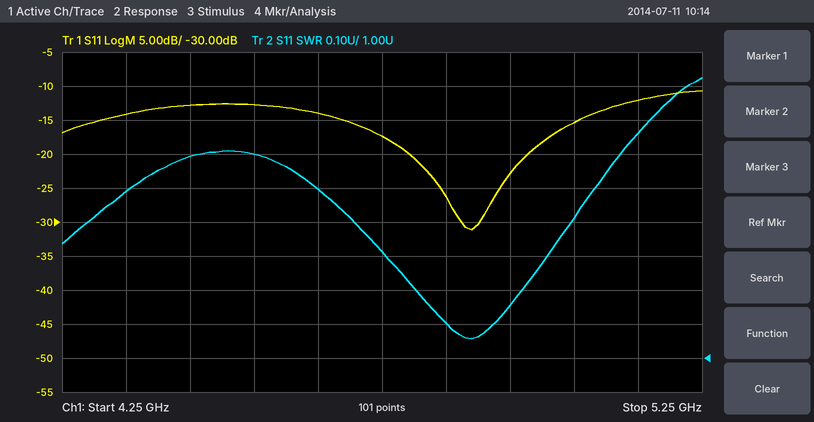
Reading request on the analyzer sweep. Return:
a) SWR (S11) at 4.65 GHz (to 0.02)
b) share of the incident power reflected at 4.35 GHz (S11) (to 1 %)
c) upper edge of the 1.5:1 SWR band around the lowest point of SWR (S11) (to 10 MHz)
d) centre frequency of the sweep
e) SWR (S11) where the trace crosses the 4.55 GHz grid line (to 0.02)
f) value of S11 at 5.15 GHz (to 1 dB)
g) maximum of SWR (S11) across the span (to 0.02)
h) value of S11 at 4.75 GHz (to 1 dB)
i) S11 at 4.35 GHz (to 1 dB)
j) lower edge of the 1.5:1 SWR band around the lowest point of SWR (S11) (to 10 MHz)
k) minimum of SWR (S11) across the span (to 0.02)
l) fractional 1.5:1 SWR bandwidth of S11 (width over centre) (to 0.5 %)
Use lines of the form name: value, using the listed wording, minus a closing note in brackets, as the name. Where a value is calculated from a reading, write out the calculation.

SWR (S11) at 4.65 GHz: 1.50
share of the incident power reflected at 4.35 GHz (S11): 10^(-14/10) ≈ 4 %
upper edge of the 1.5:1 SWR band around the lowest point of SWR (S11): 5.08 GHz
centre frequency of the sweep: 4.75 GHz
SWR (S11) where the trace crosses the 4.55 GHz grid line: 1.60
value of S11 at 5.15 GHz: -12 dB
maximum of SWR (S11) across the span: 1.82
value of S11 at 4.75 GHz: -17 dB
S11 at 4.35 GHz: -14 dB
lower edge of the 1.5:1 SWR band around the lowest point of SWR (S11): 4.65 GHz
minimum of SWR (S11) across the span: 1.06
fractional 1.5:1 SWR bandwidth of S11 (width over centre): 430 MHz / 4.865 GHz ≈ 8.84 %, so 9.0 % to the nearest 0.5 %
